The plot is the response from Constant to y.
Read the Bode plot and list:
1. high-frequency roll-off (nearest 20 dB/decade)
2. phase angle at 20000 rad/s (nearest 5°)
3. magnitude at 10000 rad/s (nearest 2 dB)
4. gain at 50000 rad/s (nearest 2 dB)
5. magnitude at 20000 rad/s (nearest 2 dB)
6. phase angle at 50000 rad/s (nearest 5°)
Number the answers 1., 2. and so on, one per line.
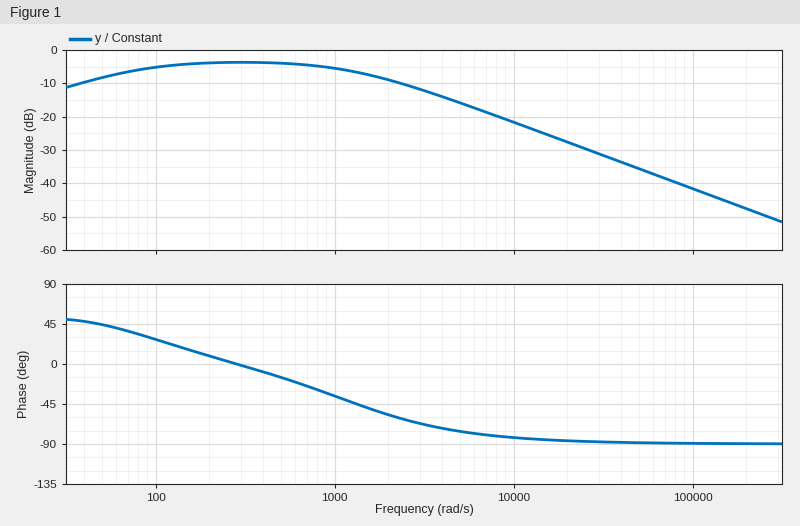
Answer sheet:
1. -20 dB/decade
2. -85°
3. -22 dB
4. -36 dB
5. -28 dB
6. -90°
